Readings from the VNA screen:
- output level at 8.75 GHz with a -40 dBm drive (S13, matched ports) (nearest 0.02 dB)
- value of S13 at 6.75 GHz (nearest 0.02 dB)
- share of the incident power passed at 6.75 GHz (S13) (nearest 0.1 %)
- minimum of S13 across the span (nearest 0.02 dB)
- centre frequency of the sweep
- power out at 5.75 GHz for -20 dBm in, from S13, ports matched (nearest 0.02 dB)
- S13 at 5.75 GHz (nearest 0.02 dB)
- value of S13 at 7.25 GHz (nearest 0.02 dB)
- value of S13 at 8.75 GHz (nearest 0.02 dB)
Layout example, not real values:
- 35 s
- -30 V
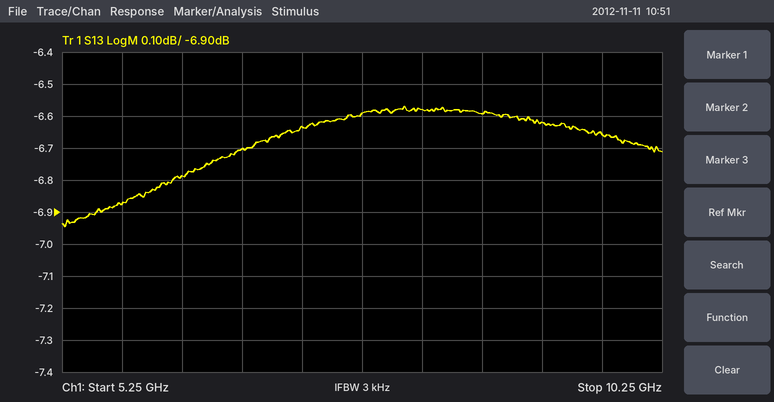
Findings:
- -46.60 dBm
- -6.70 dB
- 21.4 %
- -6.94 dB
- 7.75 GHz
- -26.88 dBm
- -6.88 dB
- -6.64 dB
- -6.60 dB
